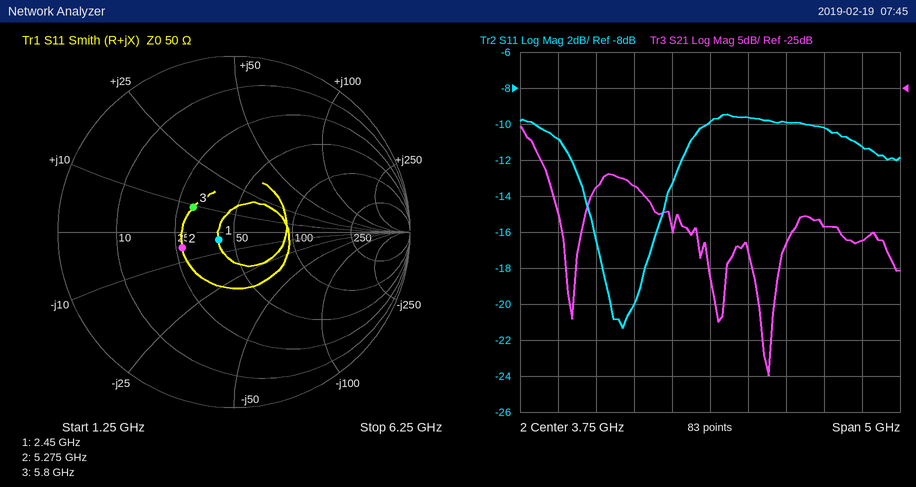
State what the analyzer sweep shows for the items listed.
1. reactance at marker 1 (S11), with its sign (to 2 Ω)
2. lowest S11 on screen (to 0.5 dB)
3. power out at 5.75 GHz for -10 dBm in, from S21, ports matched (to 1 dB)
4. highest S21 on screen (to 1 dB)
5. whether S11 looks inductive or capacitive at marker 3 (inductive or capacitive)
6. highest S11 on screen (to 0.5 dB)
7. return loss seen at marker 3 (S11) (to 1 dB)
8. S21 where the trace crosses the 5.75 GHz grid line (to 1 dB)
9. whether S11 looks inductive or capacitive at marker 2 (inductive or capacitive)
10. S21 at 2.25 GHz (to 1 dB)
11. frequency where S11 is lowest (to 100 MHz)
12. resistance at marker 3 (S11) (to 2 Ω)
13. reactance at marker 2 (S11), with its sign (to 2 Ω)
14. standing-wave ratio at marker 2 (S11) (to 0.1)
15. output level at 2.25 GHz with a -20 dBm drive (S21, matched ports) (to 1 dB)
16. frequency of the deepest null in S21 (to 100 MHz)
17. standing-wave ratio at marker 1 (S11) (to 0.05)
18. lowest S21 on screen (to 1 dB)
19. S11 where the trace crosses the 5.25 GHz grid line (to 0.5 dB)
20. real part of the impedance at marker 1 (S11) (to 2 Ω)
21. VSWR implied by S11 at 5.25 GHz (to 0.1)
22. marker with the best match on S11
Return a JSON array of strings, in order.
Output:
["-4 Ω", "-21.5 dB", "-56 dBm", "-30 dB", "inductive", "-9.5 dB", "11 dB", "-46 dB", "capacitive", "-39 dB", "2.6 GHz", "30 Ω", "-6 Ω", "1.9", "-59 dBm", "4.5 GHz", "1.20", "-65 dB", "-10.0 dB", "42 Ω", "1.9", "marker 1"]
